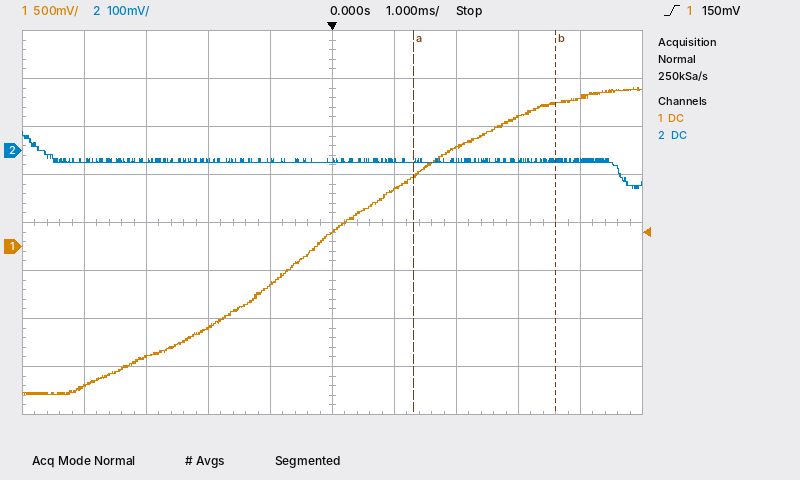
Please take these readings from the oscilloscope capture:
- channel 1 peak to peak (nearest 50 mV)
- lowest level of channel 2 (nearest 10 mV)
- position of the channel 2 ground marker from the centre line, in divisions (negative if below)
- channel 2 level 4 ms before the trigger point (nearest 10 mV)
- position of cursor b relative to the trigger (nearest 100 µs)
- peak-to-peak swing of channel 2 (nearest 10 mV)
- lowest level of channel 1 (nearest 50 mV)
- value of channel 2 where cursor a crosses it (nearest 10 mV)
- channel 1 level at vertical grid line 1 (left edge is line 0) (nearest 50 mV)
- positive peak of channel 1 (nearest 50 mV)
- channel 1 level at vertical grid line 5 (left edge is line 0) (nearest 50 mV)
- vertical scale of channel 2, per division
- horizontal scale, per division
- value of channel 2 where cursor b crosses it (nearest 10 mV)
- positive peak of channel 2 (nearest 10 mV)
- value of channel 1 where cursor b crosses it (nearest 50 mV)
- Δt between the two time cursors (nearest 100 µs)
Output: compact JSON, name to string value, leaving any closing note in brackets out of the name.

{"channel 1 peak to peak": "3.20 V", "lowest level of channel 2": "-80 mV", "position of the channel 2 ground marker from the centre line, in divisions": "+1.5 div", "channel 2 level 4 ms before the trigger point": "-20 mV", "position of cursor b relative to the trigger": "+3.6 ms", "peak-to-peak swing of channel 2": "120 mV", "lowest level of channel 1": "-1.55 V", "value of channel 2 where cursor a crosses it": "-20 mV", "channel 1 level at vertical grid line 1 (left edge is line 0)": "-1.45 V", "positive peak of channel 1": "1.65 V", "channel 1 level at vertical grid line 5 (left edge is line 0)": "150 mV", "vertical scale of channel 2, per division": "100 mV", "horizontal scale, per division": "1 ms", "value of channel 2 where cursor b crosses it": "-20 mV", "positive peak of channel 2": "40 mV", "value of channel 1 where cursor b crosses it": "1.50 V", "Δt between the two time cursors": "2.3 ms"}
